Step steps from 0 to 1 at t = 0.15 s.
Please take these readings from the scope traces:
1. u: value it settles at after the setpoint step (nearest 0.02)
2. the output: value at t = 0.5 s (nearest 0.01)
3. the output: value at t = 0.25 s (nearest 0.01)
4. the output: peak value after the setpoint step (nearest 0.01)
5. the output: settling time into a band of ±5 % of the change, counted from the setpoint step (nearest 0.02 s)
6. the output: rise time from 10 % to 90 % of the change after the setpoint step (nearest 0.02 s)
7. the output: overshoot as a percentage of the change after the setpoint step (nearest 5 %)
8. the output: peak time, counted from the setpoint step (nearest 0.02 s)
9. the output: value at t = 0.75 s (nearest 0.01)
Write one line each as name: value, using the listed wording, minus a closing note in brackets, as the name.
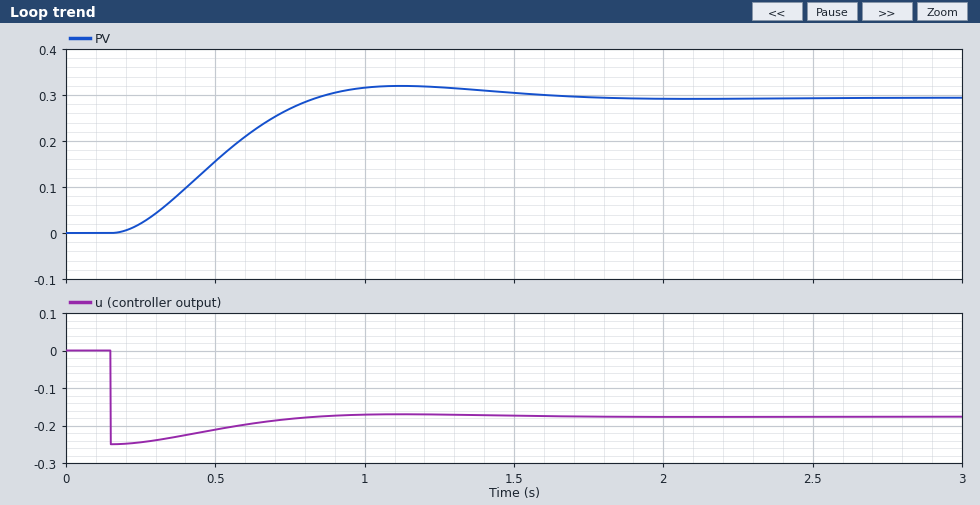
u: value it settles at after the setpoint step: -0.18
the output: value at t = 0.5 s: 0.16
the output: value at t = 0.25 s: 0.02
the output: peak value after the setpoint step: 0.32
the output: settling time into a band of ±5 % of the change, counted from the setpoint step: 1.28 s
the output: rise time from 10 % to 90 % of the change after the setpoint step: 0.46 s
the output: overshoot as a percentage of the change after the setpoint step: 10 %
the output: peak time, counted from the setpoint step: 0.98 s
the output: value at t = 0.75 s: 0.27
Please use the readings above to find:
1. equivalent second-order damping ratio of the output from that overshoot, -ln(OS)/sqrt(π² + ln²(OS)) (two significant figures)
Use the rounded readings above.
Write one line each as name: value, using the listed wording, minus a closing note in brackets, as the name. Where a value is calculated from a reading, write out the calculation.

equivalent second-order damping ratio of the output from that overshoot, -ln(OS)/sqrt(π² + ln²(OS)): ln(0.1) = -2.303; 2.303 / sqrt(9.870 + 5.302) = 0.59
